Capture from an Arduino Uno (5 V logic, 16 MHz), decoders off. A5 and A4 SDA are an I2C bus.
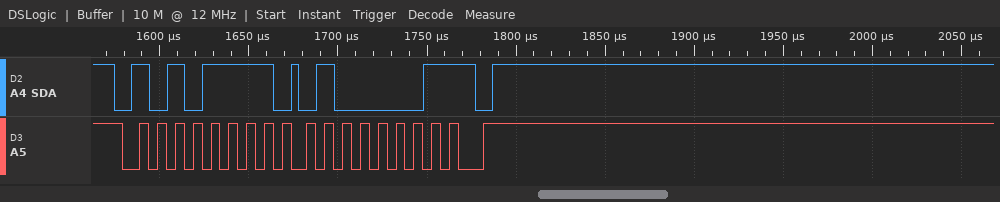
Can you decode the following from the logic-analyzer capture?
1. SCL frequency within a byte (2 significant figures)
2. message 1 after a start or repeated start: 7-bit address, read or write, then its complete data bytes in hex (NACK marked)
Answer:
100 kHz
0x57 read: 41 NACK
